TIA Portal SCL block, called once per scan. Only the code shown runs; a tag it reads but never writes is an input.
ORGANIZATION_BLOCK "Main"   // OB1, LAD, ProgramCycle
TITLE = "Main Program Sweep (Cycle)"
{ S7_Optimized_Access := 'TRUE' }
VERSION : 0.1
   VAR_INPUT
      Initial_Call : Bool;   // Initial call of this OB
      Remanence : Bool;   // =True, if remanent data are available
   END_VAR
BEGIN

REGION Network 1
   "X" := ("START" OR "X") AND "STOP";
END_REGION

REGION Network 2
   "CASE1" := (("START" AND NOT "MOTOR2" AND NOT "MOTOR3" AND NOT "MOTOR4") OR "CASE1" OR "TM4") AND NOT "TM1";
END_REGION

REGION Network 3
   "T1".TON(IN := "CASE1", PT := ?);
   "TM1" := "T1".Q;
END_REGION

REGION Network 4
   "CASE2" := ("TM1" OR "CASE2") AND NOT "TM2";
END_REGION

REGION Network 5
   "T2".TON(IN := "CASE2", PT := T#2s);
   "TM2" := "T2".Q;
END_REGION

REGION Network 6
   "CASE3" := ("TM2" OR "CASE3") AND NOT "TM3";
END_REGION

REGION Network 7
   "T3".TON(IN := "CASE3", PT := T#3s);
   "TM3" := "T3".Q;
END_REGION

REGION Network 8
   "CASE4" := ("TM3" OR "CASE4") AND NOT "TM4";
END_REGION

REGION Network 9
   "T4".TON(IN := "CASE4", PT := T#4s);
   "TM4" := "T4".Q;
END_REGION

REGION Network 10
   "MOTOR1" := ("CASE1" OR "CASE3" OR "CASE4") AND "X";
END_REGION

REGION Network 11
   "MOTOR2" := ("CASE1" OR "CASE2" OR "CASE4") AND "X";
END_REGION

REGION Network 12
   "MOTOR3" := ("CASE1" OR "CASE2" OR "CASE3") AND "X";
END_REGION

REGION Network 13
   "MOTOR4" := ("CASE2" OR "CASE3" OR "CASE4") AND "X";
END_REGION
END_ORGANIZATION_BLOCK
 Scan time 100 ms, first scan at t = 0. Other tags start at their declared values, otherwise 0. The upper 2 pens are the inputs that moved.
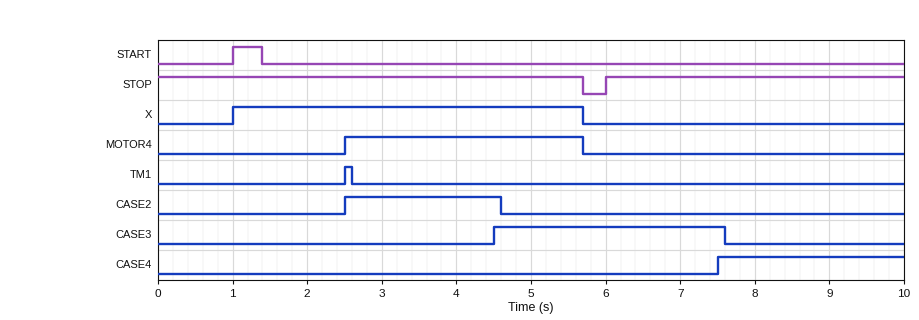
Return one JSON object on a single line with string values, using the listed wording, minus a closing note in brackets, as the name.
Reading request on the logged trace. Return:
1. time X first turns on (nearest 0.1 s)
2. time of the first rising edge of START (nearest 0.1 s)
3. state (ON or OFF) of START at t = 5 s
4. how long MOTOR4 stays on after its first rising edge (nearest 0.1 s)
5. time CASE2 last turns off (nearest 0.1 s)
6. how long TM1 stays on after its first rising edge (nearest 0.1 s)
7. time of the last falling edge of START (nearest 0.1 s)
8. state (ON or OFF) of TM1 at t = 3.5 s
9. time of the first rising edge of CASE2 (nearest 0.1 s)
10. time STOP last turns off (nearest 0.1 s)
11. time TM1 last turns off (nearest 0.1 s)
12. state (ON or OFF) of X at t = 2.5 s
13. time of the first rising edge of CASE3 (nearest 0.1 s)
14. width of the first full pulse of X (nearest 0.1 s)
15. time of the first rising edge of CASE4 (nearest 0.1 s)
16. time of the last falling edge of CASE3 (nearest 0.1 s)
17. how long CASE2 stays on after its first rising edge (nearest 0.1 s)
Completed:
{"time X first turns on": "1.0 s", "time of the first rising edge of START": "1.0 s", "state (ON or OFF) of START at t = 5 s": "OFF", "how long MOTOR4 stays on after its first rising edge": "3.2 s", "time CASE2 last turns off": "4.6 s", "how long TM1 stays on after its first rising edge": "0.1 s", "time of the last falling edge of START": "1.4 s", "state (ON or OFF) of TM1 at t = 3.5 s": "OFF", "time of the first rising edge of CASE2": "2.5 s", "time STOP last turns off": "5.7 s", "time TM1 last turns off": "2.6 s", "state (ON or OFF) of X at t = 2.5 s": "ON", "time of the first rising edge of CASE3": "4.5 s", "width of the first full pulse of X": "4.7 s", "time of the first rising edge of CASE4": "7.5 s", "time of the last falling edge of CASE3": "7.6 s", "how long CASE2 stays on after its first rising edge": "2.1 s"}
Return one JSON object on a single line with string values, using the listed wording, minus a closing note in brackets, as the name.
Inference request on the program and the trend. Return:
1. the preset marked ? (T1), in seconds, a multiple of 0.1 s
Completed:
{"the preset marked ? (T1), in seconds, a multiple of 0.1 s": "1.5 s"}
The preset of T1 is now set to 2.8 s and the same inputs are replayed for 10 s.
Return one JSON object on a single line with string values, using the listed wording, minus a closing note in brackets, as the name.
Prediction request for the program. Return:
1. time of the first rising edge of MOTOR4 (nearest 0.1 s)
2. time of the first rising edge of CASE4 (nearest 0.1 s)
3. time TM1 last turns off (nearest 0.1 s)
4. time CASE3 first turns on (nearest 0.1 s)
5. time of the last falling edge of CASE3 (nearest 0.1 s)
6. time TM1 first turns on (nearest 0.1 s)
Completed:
{"time of the first rising edge of MOTOR4": "3.8 s", "time of the first rising edge of CASE4": "8.8 s", "time TM1 last turns off": "3.9 s", "time CASE3 first turns on": "5.8 s", "time of the last falling edge of CASE3": "8.9 s", "time TM1 first turns on": "3.8 s"}
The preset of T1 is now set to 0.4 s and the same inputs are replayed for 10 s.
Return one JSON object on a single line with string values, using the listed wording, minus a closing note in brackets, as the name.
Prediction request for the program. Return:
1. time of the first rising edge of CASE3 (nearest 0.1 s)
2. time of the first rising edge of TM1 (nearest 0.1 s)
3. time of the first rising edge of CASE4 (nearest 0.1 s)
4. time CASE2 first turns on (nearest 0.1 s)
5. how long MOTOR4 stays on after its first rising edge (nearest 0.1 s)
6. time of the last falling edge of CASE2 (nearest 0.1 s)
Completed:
{"time of the first rising edge of CASE3": "3.4 s", "time of the first rising edge of TM1": "1.4 s", "time of the first rising edge of CASE4": "6.4 s", "time CASE2 first turns on": "1.4 s", "how long MOTOR4 stays on after its first rising edge": "4.3 s", "time of the last falling edge of CASE2": "3.5 s"}
